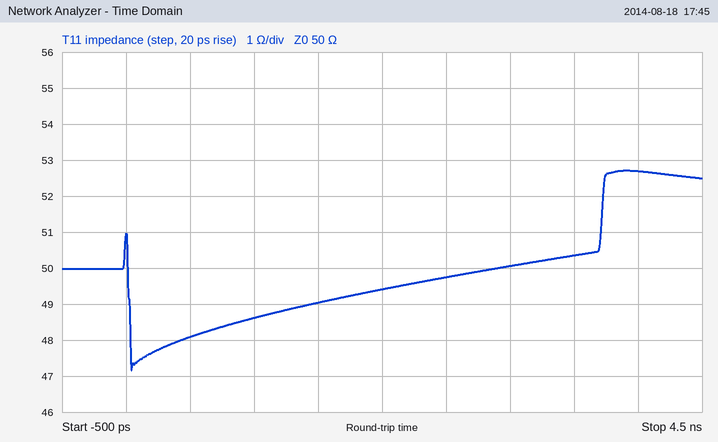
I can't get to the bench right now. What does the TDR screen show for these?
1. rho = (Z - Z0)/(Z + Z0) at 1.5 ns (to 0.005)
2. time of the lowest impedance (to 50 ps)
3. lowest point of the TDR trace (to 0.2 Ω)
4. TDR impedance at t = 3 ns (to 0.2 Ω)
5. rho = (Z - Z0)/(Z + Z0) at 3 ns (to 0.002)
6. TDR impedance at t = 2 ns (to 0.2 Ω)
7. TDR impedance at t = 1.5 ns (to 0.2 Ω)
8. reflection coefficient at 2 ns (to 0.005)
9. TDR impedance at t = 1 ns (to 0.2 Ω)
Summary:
-0.010
50 ps
47.2 Ω
50.0 Ω
0.000
49.4 Ω
49.0 Ω
-0.005
48.6 Ω
